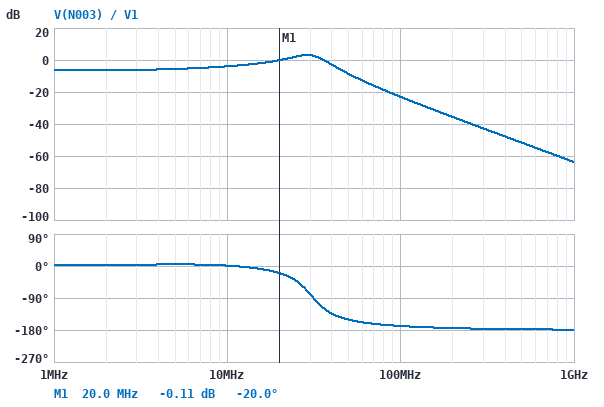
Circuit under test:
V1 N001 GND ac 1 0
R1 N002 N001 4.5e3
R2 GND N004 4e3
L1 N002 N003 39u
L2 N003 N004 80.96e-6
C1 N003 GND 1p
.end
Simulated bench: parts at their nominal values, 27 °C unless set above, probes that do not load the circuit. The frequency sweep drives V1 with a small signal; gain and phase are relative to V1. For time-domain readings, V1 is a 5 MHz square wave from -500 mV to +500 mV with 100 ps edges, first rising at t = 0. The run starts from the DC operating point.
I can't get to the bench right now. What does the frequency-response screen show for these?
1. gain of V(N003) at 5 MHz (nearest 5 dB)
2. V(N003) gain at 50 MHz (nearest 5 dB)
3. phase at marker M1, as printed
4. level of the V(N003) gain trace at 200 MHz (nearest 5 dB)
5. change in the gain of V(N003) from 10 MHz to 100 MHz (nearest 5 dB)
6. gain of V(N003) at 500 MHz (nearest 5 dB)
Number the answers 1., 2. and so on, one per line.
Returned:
1. -5 dB
2. -10 dB
3. -20.0 deg
4. -35 dB
5. -20 dB
6. -50 dB
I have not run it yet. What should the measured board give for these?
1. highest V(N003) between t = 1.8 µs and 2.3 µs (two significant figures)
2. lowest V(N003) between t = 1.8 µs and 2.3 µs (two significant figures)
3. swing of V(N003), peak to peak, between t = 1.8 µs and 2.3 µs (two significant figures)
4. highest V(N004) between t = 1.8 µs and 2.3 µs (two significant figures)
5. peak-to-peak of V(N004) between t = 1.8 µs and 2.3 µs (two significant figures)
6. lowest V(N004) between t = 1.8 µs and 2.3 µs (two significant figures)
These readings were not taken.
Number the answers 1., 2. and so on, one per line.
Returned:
1. 630 mV
2. -630 mV
3. 1.3 V
4. 240 mV
5. 480 mV
6. -240 mV
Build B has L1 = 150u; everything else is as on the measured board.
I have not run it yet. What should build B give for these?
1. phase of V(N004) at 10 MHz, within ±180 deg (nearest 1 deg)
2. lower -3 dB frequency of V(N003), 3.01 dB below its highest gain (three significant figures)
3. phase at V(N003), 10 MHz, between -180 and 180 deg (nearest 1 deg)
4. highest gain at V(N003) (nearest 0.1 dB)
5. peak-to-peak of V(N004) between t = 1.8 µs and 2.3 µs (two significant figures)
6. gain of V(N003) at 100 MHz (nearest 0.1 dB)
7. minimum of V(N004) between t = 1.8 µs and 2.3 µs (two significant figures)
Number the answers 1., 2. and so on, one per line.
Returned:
1. -70 deg
2. 17.5 MHz
3. -18 deg
4. 1.5 dB
5. 470 mV
6. -35.0 dB
7. -230 mV
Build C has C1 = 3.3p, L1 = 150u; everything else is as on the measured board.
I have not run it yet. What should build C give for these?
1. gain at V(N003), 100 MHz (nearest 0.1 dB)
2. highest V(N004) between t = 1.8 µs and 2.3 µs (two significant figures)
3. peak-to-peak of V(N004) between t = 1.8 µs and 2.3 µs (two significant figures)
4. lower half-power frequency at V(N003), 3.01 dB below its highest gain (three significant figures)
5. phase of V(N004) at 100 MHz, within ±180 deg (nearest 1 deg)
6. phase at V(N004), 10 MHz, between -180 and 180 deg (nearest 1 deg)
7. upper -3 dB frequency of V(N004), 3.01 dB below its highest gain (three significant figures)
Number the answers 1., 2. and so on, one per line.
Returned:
1. -45.7 dB
2. 250 mV
3. 510 mV
4. 5.51 MHz
5. 97 deg
6. -116 deg
7. 12.7 MHz
